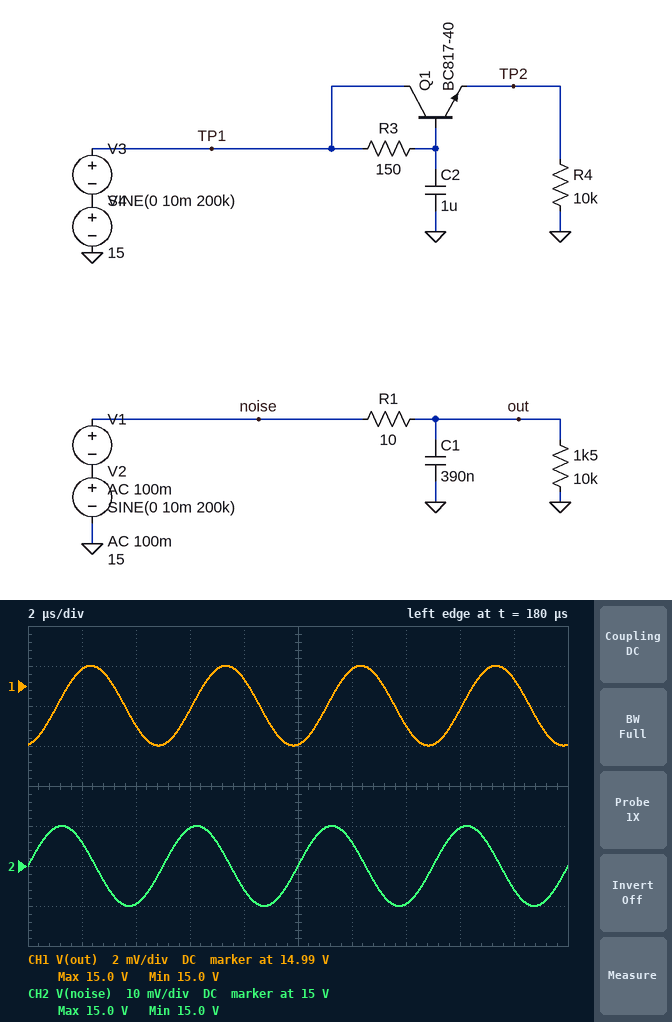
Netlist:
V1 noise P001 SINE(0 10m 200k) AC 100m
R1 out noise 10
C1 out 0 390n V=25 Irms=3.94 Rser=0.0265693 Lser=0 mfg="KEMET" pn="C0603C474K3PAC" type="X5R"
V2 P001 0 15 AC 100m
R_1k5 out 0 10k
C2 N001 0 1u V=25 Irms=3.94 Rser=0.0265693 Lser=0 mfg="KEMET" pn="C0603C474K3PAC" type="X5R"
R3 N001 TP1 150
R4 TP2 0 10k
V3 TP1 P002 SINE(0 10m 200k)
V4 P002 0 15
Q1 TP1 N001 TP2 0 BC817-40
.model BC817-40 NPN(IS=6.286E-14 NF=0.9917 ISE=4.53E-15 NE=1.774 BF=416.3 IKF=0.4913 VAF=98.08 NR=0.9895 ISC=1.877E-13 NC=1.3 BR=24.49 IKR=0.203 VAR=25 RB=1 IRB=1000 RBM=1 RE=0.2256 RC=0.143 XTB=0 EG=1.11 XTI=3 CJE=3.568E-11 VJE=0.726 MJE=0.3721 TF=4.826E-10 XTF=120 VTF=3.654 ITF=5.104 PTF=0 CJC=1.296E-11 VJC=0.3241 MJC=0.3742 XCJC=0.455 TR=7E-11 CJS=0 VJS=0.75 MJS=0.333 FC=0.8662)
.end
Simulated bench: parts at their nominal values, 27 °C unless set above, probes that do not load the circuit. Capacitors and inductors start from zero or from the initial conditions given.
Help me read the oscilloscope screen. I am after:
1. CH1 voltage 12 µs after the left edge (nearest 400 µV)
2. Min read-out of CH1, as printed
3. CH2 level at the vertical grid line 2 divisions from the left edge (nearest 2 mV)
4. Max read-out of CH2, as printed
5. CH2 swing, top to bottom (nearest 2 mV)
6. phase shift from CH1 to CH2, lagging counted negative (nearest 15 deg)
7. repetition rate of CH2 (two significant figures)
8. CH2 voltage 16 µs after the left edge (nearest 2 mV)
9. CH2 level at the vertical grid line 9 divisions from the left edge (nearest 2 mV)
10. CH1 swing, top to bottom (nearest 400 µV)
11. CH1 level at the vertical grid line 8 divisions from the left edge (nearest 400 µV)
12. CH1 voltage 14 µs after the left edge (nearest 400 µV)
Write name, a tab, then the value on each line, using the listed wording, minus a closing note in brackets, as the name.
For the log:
CH1 voltage 12 µs after the left edge	14.9868 V
Min read-out of CH1, as printed	15.0 V
CH2 level at the vertical grid line 2 divisions from the left edge	14.990 V
Max read-out of CH2, as printed	15.0 V
CH2 swing, top to bottom	20 mV
phase shift from CH1 to CH2, lagging counted negative	75 deg
repetition rate of CH2	200 kHz
CH2 voltage 16 µs after the left edge	15.010 V
CH2 level at the vertical grid line 9 divisions from the left edge	14.994 V
CH1 swing, top to bottom	4.0 mV
CH1 level at the vertical grid line 8 divisions from the left edge	14.9848 V
CH1 voltage 14 µs after the left edge	14.9840 V
